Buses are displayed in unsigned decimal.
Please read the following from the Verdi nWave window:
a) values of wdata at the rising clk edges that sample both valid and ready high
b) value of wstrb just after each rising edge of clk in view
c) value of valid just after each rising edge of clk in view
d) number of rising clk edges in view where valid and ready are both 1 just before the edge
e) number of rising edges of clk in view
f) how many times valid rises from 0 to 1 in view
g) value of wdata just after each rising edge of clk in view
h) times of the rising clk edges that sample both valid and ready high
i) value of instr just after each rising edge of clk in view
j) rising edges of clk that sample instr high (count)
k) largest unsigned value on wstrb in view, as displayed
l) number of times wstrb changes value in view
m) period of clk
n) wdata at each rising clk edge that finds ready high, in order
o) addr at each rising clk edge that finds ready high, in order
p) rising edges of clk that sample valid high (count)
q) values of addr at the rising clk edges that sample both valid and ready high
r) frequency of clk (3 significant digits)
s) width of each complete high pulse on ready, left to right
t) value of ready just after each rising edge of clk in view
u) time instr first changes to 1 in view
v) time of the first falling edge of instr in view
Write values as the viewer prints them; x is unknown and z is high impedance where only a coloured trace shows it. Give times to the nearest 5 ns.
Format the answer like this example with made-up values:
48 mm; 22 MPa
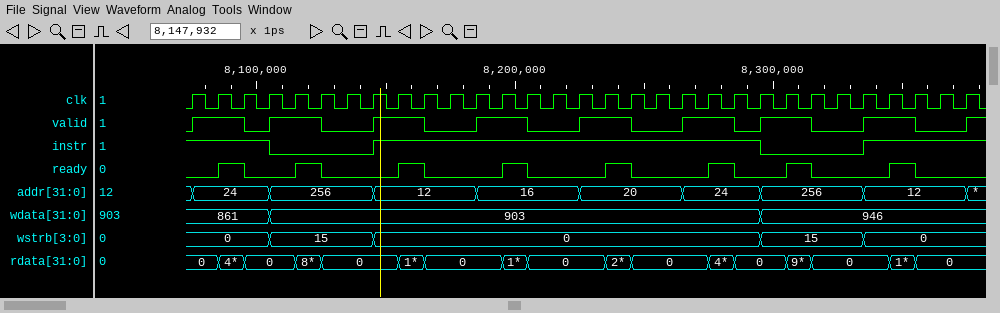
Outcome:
861, 903, 903, 903, 903, 903, 946, 946; 0, 0, 0, 15, 15, 15, 15, 0, 0, 0, 0, 0, 0, 0, 0, 0, 0, 0, 0, 0, 0, 0, 15, 15, 15, 15, 0, 0, 0, 0, 0; 1 1 0 1 1 0 0 1 1 0 0 1 1 0 0 1 1 0 0 1 1 0 1 1 0 0 1 1 0 0 1; 8; 31; 9; 861, 861, 861, 903, 903, 903, 903, 903, 903, 903, 903, 903, 903, 903, 903, 903, 903, 903, 903, 903, 903, 903, 946, 946, 946, 946, 946, 946, 946, 946, 946; 8095 ns, 8125 ns, 8165 ns, 8205 ns, 8245 ns, 8285 ns, 8315 ns, 8355 ns; 1 1 1 0 0 0 0 1 1 1 1 1 1 1 1 1 1 1 1 1 1 1 0 0 0 0 1 1 1 1 1; 23; 15; 4; 10 ns; 861, 903, 903, 903, 903, 903, 946, 946; 24, 256, 12, 16, 20, 24, 256, 12; 16; 24, 256, 12, 16, 20, 24, 256, 12; 100 MHz; 10 ns, 10 ns, 10 ns, 10 ns, 10 ns, 10 ns, 10 ns, 10 ns; 0 1 0 0 1 0 0 0 1 0 0 0 1 0 0 0 1 0 0 0 1 0 0 1 0 0 0 1 0 0 0; 8145 ns; 8105 ns
